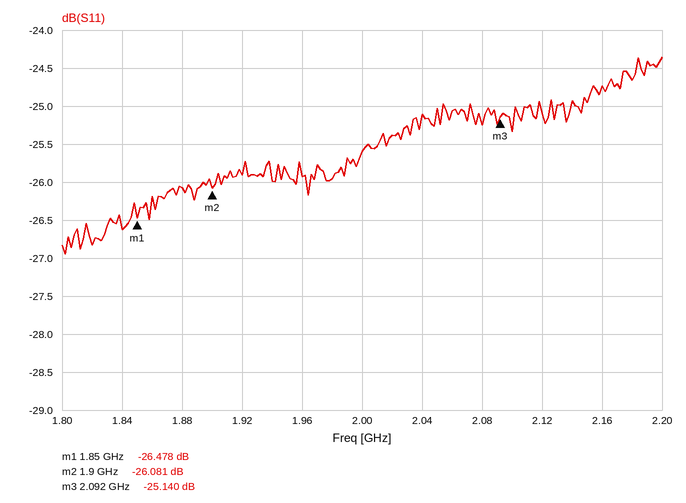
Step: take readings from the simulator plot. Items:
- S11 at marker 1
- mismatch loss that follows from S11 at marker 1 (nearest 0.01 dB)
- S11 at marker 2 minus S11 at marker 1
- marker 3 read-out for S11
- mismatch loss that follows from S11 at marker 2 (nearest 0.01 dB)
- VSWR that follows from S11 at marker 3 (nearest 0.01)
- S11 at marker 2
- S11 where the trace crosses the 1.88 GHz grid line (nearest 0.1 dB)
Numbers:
-26.478 dB
0.01 dB
0.397 dB
-25.140 dB
0.01 dB
1.12
-26.081 dB
-26.1 dB
